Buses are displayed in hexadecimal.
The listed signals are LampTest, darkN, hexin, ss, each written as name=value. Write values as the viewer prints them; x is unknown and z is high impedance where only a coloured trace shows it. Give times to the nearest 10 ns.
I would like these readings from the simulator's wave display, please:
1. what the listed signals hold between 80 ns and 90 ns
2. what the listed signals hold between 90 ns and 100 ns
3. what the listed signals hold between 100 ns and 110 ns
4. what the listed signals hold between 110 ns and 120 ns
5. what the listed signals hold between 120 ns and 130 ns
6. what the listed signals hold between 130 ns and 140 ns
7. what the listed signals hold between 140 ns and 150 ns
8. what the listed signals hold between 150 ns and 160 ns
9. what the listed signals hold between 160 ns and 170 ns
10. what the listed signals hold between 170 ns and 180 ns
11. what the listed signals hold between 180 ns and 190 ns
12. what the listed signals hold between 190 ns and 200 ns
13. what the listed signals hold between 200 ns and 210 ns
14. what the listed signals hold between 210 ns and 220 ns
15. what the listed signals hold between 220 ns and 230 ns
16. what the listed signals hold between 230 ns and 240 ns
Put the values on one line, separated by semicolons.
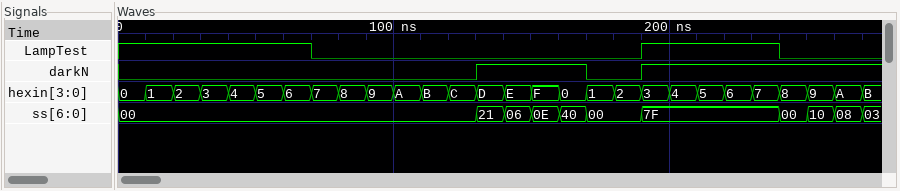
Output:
LampTest=0, darkN=0, hexin=8, ss=00; LampTest=0, darkN=0, hexin=9, ss=00; LampTest=0, darkN=0, hexin=A, ss=00; LampTest=0, darkN=0, hexin=B, ss=00; LampTest=0, darkN=0, hexin=C, ss=00; LampTest=0, darkN=1, hexin=D, ss=21; LampTest=0, darkN=1, hexin=E, ss=06; LampTest=0, darkN=1, hexin=F, ss=0E; LampTest=0, darkN=1, hexin=0, ss=40; LampTest=0, darkN=0, hexin=1, ss=00; LampTest=0, darkN=0, hexin=2, ss=00; LampTest=1, darkN=1, hexin=3, ss=7F; LampTest=1, darkN=1, hexin=4, ss=7F; LampTest=1, darkN=1, hexin=5, ss=7F; LampTest=1, darkN=1, hexin=6, ss=7F; LampTest=1, darkN=1, hexin=7, ss=7F
